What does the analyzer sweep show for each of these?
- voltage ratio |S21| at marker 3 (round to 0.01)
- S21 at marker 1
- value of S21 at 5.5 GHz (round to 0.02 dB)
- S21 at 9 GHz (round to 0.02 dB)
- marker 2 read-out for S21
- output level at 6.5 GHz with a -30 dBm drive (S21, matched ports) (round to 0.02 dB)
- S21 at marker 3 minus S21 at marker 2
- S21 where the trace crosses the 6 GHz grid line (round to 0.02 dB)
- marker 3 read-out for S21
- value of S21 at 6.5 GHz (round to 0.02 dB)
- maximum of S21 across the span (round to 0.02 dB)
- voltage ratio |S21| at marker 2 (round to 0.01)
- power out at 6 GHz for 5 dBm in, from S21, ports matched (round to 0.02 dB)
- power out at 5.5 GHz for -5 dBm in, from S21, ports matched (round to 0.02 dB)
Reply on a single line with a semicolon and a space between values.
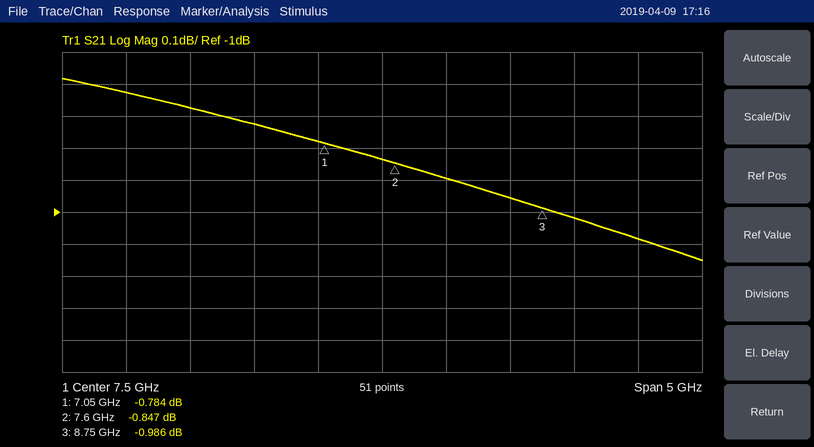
0.89; -0.784 dB; -0.62 dB; -1.02 dB; -0.847 dB; -30.72 dBm; -0.139 dB; -0.68 dB; -0.986 dB; -0.72 dB; -0.58 dB; 0.91; 4.32 dBm; -5.62 dBm
